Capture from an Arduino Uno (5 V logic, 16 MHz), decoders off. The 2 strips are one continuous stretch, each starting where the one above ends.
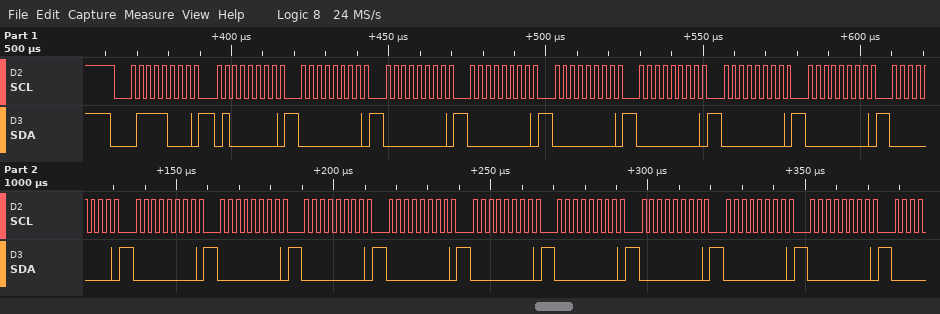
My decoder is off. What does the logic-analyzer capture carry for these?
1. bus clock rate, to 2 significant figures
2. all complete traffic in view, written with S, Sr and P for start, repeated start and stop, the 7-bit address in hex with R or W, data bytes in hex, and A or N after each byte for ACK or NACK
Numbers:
400 kHz
S 3CW A 40 A 00 A 00 A 00 A 00 A 00 A 00 A 00 A 00 A 00 A 00 A 00 A 00 A 00 A 00 A 00 A 00 A 00 A
